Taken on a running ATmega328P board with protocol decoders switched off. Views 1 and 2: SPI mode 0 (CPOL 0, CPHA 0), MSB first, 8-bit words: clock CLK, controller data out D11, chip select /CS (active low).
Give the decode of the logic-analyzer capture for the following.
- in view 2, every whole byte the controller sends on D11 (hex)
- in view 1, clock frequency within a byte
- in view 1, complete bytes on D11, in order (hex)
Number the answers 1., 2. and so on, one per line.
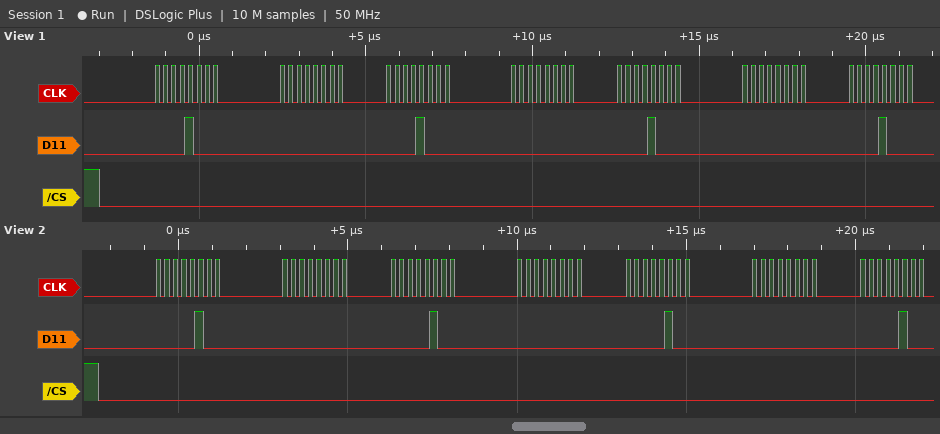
1. 0x04 0x00 0x04 0x00 0x04 0x00 0x04
2. 4 MHz
3. 08 00 08 00 08 00 08
